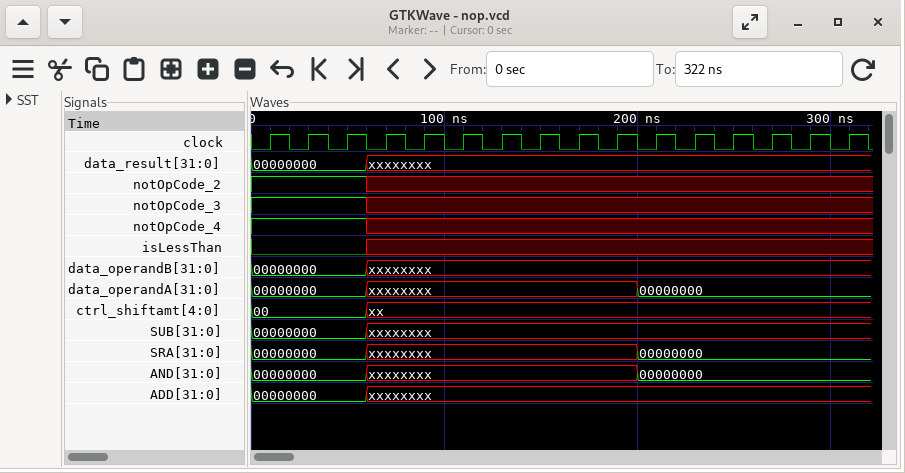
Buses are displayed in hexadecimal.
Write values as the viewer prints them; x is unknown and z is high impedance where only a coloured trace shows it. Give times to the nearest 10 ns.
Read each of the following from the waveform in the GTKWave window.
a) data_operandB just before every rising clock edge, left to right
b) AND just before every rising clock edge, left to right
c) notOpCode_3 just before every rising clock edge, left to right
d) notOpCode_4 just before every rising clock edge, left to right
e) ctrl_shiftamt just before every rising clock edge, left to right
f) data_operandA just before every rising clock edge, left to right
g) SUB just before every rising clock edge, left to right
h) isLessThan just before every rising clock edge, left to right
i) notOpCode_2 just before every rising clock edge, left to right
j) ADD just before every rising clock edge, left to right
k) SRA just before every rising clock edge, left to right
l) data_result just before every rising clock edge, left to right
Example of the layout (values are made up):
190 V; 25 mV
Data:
00000000, 00000000, 00000000, xxxxxxxx, xxxxxxxx, xxxxxxxx, xxxxxxxx, xxxxxxxx, xxxxxxxx, xxxxxxxx, xxxxxxxx, xxxxxxxx, xxxxxxxx, xxxxxxxx, xxxxxxxx, xxxxxxxx; 00000000, 00000000, 00000000, xxxxxxxx, xxxxxxxx, xxxxxxxx, xxxxxxxx, xxxxxxxx, xxxxxxxx, xxxxxxxx, 00000000, 00000000, 00000000, 00000000, 00000000, 00000000; 1 1 1 x x x x x x x x x x x x x; 1 1 1 x x x x x x x x x x x x x; 00, 00, 00, xx, xx, xx, xx, xx, xx, xx, xx, xx, xx, xx, xx, xx; 00000000, 00000000, 00000000, xxxxxxxx, xxxxxxxx, xxxxxxxx, xxxxxxxx, xxxxxxxx, xxxxxxxx, xxxxxxxx, 00000000, 00000000, 00000000, 00000000, 00000000, 00000000; 00000000, 00000000, 00000000, xxxxxxxx, xxxxxxxx, xxxxxxxx, xxxxxxxx, xxxxxxxx, xxxxxxxx, xxxxxxxx, xxxxxxxx, xxxxxxxx, xxxxxxxx, xxxxxxxx, xxxxxxxx, xxxxxxxx; 0 0 0 x x x x x x x x x x x x x; 1 1 1 x x x x x x x x x x x x x; 00000000, 00000000, 00000000, xxxxxxxx, xxxxxxxx, xxxxxxxx, xxxxxxxx, xxxxxxxx, xxxxxxxx, xxxxxxxx, xxxxxxxx, xxxxxxxx, xxxxxxxx, xxxxxxxx, xxxxxxxx, xxxxxxxx; 00000000, 00000000, 00000000, xxxxxxxx, xxxxxxxx, xxxxxxxx, xxxxxxxx, xxxxxxxx, xxxxxxxx, xxxxxxxx, 00000000, 00000000, 00000000, 00000000, 00000000, 00000000; 00000000, 00000000, 00000000, xxxxxxxx, xxxxxxxx, xxxxxxxx, xxxxxxxx, xxxxxxxx, xxxxxxxx, xxxxxxxx, xxxxxxxx, xxxxxxxx, xxxxxxxx, xxxxxxxx, xxxxxxxx, xxxxxxxx
